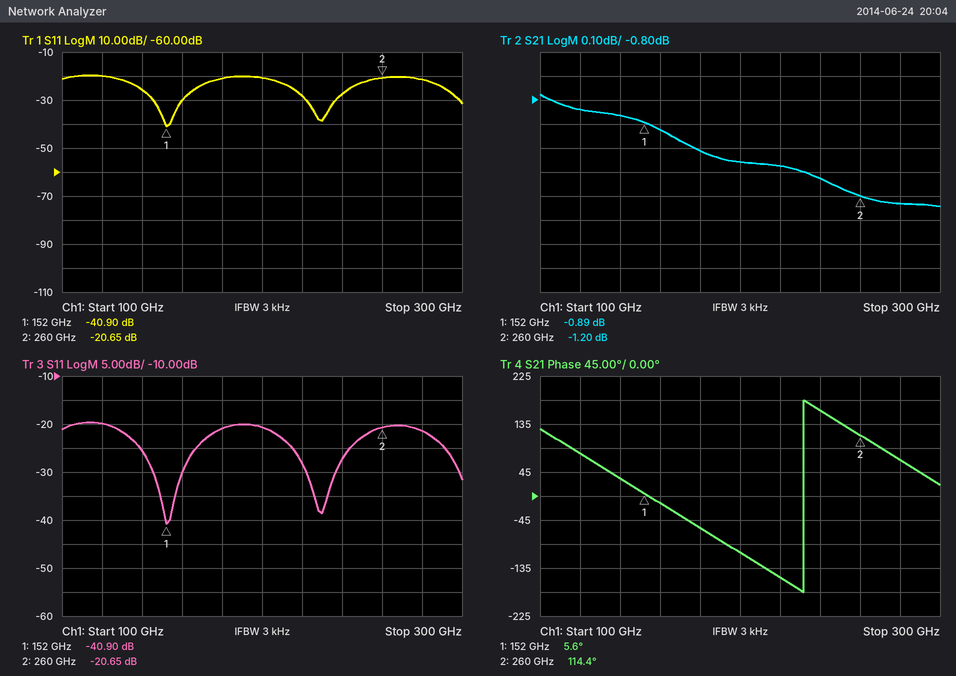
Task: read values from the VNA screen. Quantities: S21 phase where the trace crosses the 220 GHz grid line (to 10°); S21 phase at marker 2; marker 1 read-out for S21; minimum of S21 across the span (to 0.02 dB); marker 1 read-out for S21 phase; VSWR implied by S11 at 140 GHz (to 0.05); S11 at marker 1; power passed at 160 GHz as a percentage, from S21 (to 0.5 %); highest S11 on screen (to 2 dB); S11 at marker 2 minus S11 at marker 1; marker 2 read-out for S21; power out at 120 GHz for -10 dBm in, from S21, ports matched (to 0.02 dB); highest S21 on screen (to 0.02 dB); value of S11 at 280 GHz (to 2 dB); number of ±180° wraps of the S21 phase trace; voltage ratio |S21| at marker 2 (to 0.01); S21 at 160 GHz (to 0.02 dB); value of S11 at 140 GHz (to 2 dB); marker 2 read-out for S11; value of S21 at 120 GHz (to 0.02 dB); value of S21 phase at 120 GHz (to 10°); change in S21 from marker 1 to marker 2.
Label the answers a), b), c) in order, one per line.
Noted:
a) -150°
b) 114.4°
c) -0.89 dB
d) -1.24 dB
e) 5.6°
f) 1.10
g) -40.90 dB
h) 81.0 %
i) -20 dB
j) 20.25 dB
k) -1.20 dB
l) -10.84 dBm
m) -0.78 dB
n) -22 dB
o) 1
p) 0.87
q) -0.92 dB
r) -26 dB
s) -20.65 dB
t) -0.84 dB
u) 80°
v) -0.31 dB
